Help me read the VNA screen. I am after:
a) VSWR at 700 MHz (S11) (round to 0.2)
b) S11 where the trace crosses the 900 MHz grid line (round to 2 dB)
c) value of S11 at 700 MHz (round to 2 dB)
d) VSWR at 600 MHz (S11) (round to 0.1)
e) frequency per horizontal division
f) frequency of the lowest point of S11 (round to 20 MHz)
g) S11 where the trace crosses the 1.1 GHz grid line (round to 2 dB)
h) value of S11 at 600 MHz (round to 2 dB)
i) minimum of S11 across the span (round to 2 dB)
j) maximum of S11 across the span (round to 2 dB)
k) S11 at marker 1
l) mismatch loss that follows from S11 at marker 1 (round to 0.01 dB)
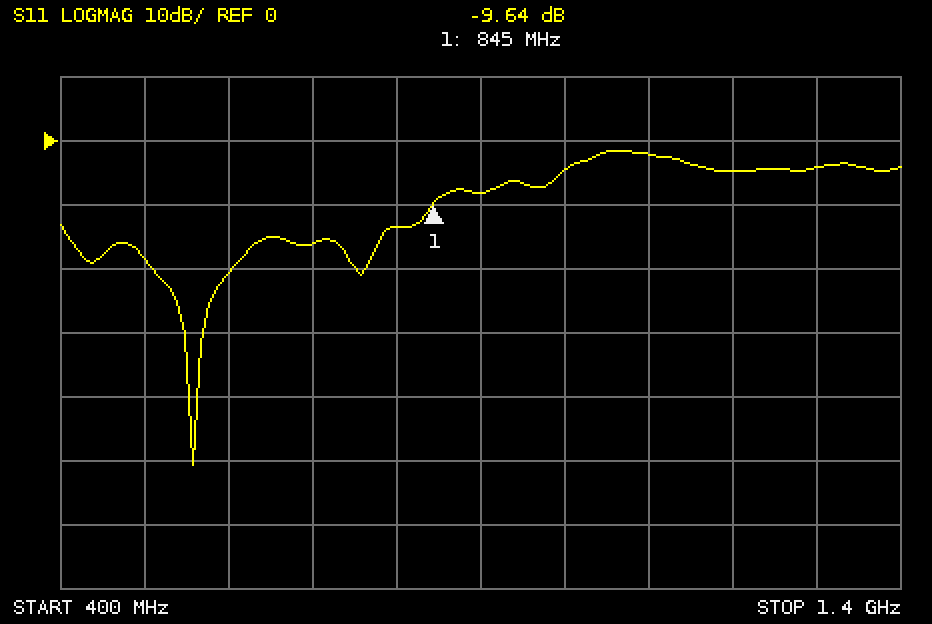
1.4
-8 dB
-16 dB
1.2
100 MHz
560 MHz
-2 dB
-20 dB
-50 dB
-2 dB
-9.64 dB
0.50 dB
